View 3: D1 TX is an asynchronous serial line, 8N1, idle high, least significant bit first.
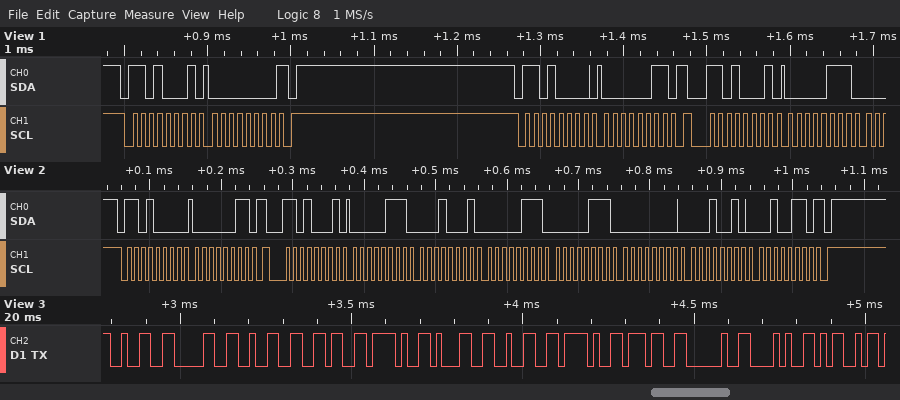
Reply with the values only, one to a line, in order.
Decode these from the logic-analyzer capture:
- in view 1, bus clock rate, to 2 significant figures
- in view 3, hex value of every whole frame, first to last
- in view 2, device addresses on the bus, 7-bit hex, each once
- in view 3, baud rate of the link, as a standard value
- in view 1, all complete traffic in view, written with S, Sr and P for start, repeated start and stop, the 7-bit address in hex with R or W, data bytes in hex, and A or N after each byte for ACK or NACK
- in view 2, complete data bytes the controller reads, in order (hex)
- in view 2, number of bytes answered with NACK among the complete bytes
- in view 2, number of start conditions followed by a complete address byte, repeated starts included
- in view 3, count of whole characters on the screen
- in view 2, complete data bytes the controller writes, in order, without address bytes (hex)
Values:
100 kHz
32 30 32 36 2F 31 32 2F 37 20 28 4D
0x68
57600 baud
S 68R A 00 N P S 68W A 03 A Sr 68R A 07 A
07 11 07 07 00 12 26
1
2
12
03
